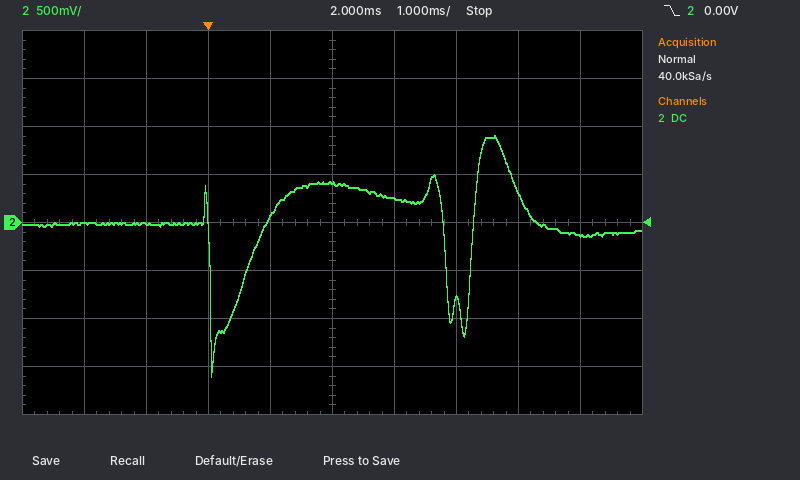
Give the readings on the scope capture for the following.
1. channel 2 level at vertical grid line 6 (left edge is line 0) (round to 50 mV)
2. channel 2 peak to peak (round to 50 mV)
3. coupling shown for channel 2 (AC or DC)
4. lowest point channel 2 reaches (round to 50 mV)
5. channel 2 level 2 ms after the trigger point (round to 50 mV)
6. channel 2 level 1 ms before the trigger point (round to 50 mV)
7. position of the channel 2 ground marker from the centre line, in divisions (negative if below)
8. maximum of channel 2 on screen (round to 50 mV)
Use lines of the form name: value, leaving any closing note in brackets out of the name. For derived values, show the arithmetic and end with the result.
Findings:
channel 2 level at vertical grid line 6 (left edge is line 0): 250 mV
channel 2 peak to peak: 900 mV − (-1.60 V) = 2.50 V
coupling shown for channel 2: DC
lowest point channel 2 reaches: -1.60 V
channel 2 level 2 ms after the trigger point: 400 mV
channel 2 level 1 ms before the trigger point: 0 mV
position of the channel 2 ground marker from the centre line, in divisions: 0.0 div
maximum of channel 2 on screen: 900 mV
